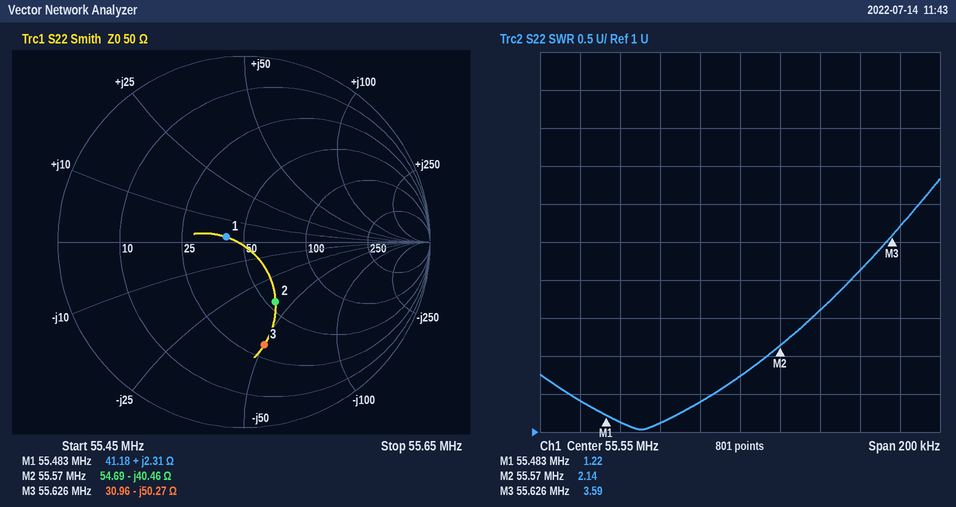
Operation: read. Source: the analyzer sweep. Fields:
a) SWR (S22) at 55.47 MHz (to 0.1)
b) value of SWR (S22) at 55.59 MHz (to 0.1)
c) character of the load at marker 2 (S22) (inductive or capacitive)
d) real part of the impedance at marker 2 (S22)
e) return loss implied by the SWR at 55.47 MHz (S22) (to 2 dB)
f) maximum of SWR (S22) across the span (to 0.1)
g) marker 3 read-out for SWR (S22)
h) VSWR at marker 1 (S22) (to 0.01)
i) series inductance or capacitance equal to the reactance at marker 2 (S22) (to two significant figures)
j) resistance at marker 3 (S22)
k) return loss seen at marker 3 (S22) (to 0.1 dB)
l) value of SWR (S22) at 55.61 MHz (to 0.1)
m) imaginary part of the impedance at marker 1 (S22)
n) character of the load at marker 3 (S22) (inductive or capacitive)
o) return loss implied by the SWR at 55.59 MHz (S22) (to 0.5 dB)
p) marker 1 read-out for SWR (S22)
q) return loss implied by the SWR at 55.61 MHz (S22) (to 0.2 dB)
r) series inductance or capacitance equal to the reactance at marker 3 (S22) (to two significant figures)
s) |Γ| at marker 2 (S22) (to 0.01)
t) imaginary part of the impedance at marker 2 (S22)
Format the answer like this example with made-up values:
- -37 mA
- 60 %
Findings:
- 1.4
- 2.6
- capacitive
- 54.69 Ω
- 16 dB
- 4.3
- 3.59
- 1.22
- 71 pF
- 30.96 Ω
- 5.0 dB
- 3.1
- +2.31 Ω
- capacitive
- 7.0 dB
- 1.22
- 5.8 dB
- 57 pF
- 0.36
- -40.46 Ω
